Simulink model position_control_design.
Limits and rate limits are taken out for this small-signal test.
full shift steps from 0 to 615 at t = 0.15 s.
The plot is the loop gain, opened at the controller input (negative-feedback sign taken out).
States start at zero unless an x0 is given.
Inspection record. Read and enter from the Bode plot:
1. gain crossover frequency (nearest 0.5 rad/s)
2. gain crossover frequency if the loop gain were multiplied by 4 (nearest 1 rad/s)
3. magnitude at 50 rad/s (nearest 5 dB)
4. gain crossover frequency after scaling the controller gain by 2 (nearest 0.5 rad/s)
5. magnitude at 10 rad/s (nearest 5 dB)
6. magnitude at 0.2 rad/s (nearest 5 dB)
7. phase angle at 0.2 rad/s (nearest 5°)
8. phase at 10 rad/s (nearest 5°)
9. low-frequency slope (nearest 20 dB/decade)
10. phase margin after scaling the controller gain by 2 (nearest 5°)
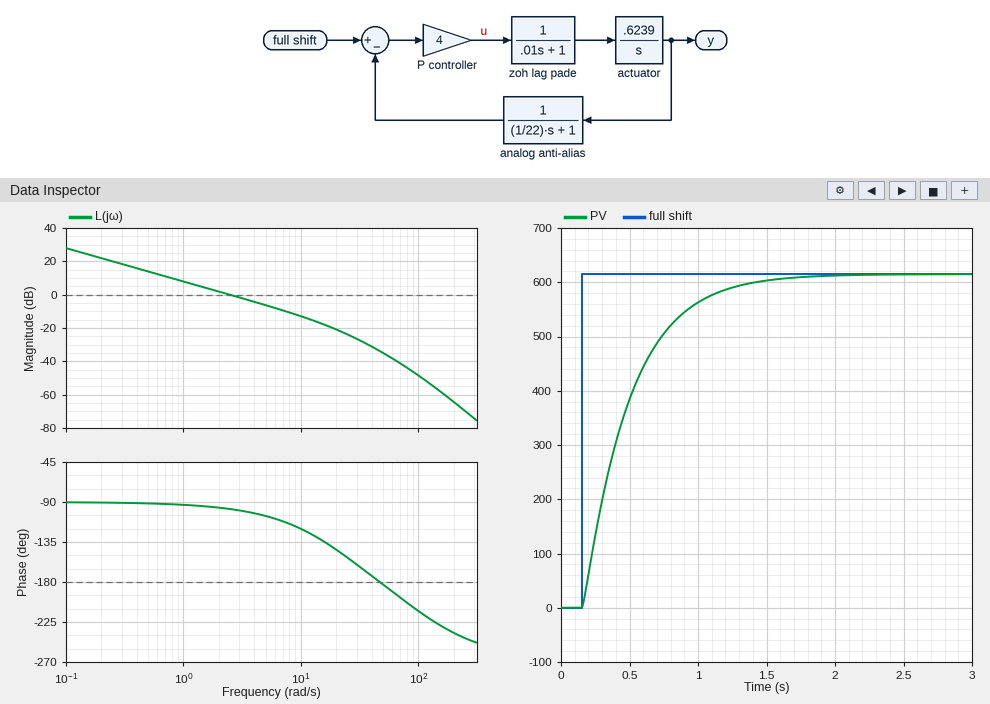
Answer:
2.5 rad/s
9 rad/s
-35 dB
5.0 rad/s
-15 dB
20 dB
-90°
-120°
-20 dB/decade
75°
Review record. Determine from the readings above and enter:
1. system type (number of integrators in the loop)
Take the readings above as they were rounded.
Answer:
1
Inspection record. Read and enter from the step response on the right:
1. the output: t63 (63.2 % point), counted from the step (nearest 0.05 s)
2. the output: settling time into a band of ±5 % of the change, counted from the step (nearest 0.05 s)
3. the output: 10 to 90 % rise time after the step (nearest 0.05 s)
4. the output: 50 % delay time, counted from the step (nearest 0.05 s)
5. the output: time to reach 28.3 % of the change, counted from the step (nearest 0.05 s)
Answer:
0.35 s
1.05 s
0.75 s
0.25 s
0.15 s
